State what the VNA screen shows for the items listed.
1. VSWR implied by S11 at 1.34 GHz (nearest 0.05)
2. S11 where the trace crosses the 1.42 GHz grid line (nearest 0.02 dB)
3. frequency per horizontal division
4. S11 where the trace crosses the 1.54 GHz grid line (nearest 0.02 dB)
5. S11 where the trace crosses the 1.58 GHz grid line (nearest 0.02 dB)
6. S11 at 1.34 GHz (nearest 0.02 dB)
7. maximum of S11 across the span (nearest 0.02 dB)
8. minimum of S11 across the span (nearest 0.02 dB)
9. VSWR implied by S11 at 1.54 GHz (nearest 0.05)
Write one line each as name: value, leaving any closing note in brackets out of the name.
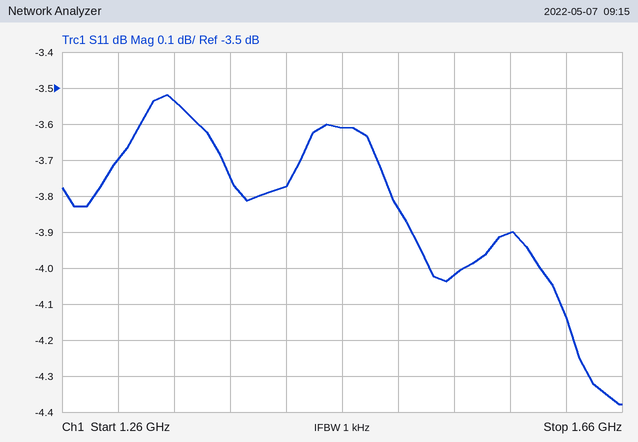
VSWR implied by S11 at 1.34 GHz: 5.00
S11 where the trace crosses the 1.42 GHz grid line: -3.78 dB
frequency per horizontal division: 40 MHz
S11 where the trace crosses the 1.54 GHz grid line: -4.02 dB
S11 where the trace crosses the 1.58 GHz grid line: -3.90 dB
S11 at 1.34 GHz: -3.54 dB
maximum of S11 across the span: -3.52 dB
minimum of S11 across the span: -4.38 dB
VSWR implied by S11 at 1.54 GHz: 4.40
